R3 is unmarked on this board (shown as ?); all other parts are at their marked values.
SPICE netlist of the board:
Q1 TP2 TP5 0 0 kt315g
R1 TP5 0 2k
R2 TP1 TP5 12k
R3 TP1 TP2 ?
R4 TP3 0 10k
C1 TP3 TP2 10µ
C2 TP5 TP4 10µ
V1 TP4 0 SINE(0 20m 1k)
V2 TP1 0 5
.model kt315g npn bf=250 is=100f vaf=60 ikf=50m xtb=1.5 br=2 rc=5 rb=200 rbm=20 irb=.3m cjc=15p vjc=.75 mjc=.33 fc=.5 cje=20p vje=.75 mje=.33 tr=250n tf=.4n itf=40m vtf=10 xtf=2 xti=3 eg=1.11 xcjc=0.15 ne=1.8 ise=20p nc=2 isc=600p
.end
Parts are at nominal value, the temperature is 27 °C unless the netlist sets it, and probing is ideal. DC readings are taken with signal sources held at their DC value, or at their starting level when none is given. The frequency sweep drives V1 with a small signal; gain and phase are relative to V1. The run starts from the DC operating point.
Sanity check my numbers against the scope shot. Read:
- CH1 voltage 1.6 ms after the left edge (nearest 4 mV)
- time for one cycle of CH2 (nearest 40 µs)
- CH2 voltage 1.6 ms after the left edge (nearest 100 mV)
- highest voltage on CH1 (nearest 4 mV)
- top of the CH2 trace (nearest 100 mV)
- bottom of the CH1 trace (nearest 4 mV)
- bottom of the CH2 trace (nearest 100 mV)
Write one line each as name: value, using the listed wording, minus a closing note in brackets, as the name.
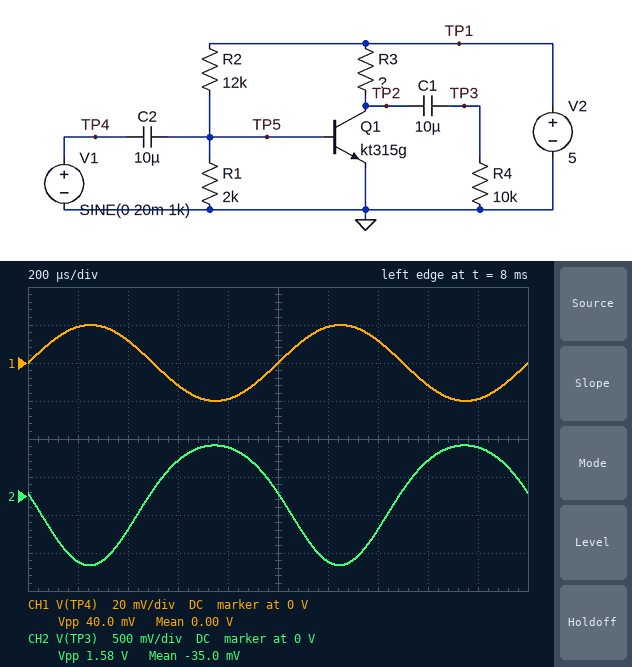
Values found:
CH1 voltage 1.6 ms after the left edge: -12 mV
time for one cycle of CH2: 1.00 ms
CH2 voltage 1.6 ms after the left edge: 500 mV
highest voltage on CH1: 20 mV
top of the CH2 trace: 700 mV
bottom of the CH1 trace: -20 mV
bottom of the CH2 trace: -900 mV
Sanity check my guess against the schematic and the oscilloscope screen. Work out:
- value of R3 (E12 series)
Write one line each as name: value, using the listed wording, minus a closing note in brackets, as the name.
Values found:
value of R3: 270 Ω
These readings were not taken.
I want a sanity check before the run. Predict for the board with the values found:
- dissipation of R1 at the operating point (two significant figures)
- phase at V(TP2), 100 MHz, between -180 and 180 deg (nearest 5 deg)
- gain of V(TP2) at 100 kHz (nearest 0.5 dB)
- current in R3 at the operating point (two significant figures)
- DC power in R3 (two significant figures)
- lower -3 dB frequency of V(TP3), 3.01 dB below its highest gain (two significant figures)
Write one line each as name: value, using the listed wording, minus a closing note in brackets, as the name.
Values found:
dissipation of R1 at the operating point: 210 µW
phase at V(TP2), 100 MHz, between -180 and 180 deg: 50 deg
gain of V(TP2) at 100 kHz: 32.0 dB
current in R3 at the operating point: 5.2 mA
DC power in R3: 7.2 mW
lower -3 dB frequency of V(TP3), 3.01 dB below its highest gain: 26 Hz
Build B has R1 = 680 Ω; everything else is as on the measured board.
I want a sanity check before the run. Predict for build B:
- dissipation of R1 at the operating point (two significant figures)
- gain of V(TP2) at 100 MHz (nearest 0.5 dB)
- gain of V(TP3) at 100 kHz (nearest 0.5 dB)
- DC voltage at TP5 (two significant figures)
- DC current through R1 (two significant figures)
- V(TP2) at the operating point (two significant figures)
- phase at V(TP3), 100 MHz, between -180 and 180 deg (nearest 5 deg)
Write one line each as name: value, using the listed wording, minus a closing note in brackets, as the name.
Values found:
dissipation of R1 at the operating point: 110 µW
gain of V(TP2) at 100 MHz: -3.5 dB
gain of V(TP3) at 100 kHz: -58.0 dB
DC voltage at TP5: 270 mV
DC current through R1: 390 µA
V(TP2) at the operating point: 5.0 V
phase at V(TP3), 100 MHz, between -180 and 180 deg: 35 deg
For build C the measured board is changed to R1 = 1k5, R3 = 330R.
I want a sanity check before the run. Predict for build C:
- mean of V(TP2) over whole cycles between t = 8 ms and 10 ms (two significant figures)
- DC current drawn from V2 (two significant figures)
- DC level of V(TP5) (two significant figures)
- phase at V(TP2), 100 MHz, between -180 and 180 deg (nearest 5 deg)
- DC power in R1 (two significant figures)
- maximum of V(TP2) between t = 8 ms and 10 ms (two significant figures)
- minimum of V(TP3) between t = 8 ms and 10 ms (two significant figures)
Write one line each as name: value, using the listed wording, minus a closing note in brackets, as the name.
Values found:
mean of V(TP2) over whole cycles between t = 8 ms and 10 ms: 4.9 V
DC current drawn from V2: 560 µA
DC level of V(TP5): 550 mV
phase at V(TP2), 100 MHz, between -180 and 180 deg: 35 deg
DC power in R1: 200 µW
maximum of V(TP2) between t = 8 ms and 10 ms: 5.0 V
minimum of V(TP3) between t = 8 ms and 10 ms: -65 mV
